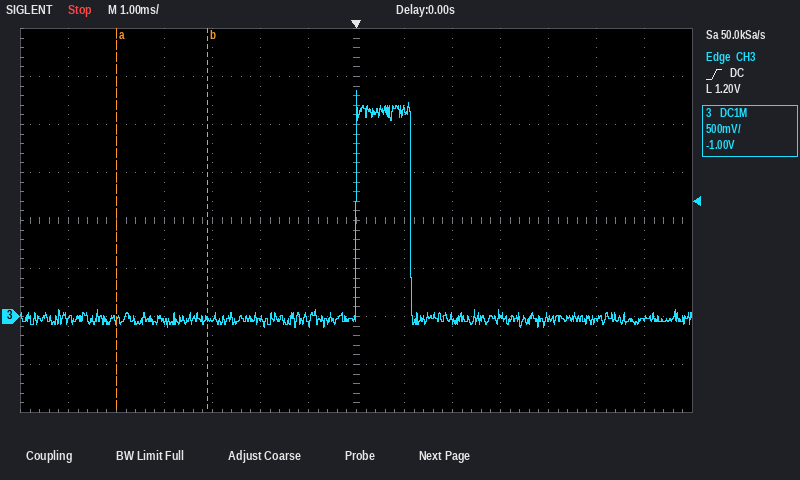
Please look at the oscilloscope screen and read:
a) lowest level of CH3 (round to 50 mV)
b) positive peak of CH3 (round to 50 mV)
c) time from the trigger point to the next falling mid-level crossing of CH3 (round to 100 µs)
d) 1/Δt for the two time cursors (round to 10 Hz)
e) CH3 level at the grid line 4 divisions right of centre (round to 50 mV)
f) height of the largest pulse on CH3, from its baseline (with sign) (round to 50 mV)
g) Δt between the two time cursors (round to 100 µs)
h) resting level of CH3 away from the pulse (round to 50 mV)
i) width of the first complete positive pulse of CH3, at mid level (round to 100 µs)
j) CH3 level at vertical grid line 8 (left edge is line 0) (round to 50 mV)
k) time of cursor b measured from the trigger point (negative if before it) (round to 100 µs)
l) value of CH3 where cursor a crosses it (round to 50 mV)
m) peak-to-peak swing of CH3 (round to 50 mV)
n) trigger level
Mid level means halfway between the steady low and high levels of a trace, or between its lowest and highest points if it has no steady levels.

-100 mV
2.35 V
1.1 ms
530 Hz
0 mV
+2.40 V
1.9 ms
-50 mV
1.1 ms
2.15 V
-3.1 ms
-50 mV
2.45 V
1.20 V
